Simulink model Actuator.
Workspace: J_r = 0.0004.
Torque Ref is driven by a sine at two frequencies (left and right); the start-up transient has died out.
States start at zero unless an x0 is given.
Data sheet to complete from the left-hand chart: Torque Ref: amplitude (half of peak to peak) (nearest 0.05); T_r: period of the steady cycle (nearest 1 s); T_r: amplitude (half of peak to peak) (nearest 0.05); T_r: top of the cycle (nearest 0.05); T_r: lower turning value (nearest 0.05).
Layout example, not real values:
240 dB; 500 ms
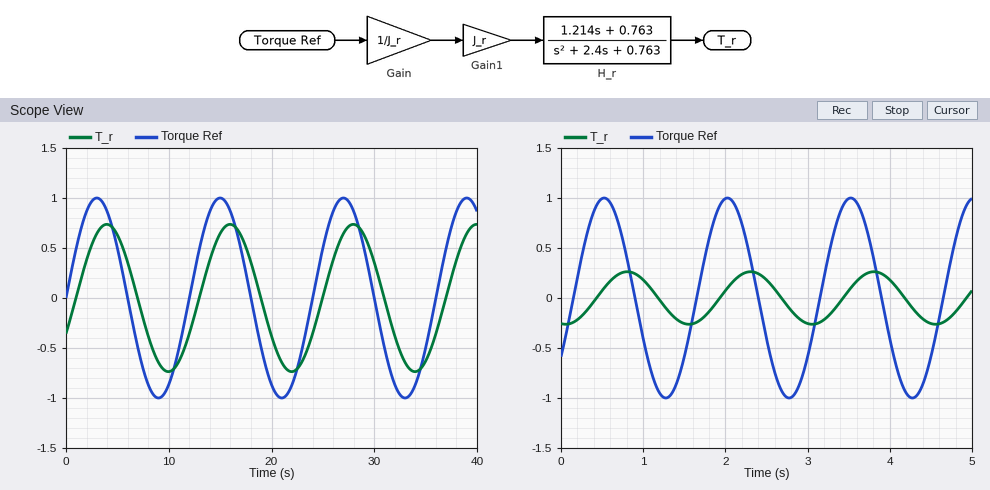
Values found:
1.00; 12 s; 0.75; 0.75; -0.75
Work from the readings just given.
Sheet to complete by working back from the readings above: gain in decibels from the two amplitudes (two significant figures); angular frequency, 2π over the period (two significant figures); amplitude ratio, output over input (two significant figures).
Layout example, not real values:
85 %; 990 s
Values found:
-2.5 dB; 0.52 rad/s; 0.75
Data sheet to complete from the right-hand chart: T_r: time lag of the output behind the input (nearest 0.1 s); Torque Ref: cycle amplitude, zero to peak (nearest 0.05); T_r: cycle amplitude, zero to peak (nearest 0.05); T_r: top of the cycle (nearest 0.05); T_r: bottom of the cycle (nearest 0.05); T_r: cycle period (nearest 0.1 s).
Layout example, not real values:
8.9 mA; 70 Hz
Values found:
0.3 s; 1.00; 0.25; 0.25; -0.25; 1.5 s
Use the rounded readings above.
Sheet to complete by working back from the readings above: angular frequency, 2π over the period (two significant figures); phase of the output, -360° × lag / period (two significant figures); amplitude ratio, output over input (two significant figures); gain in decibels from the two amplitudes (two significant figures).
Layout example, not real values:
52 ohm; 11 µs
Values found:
4.2 rad/s; -72°; 0.25; -12 dB
